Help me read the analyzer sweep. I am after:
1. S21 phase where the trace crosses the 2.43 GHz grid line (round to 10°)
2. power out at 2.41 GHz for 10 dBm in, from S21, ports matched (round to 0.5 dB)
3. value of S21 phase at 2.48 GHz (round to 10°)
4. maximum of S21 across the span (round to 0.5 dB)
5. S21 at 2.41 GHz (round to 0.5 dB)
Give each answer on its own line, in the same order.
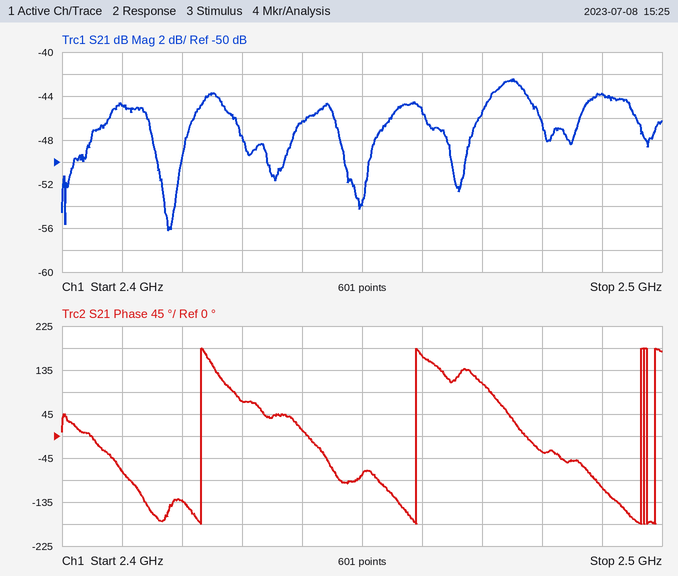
70°
-35.0 dBm
-30°
-42.5 dB
-45.0 dB
